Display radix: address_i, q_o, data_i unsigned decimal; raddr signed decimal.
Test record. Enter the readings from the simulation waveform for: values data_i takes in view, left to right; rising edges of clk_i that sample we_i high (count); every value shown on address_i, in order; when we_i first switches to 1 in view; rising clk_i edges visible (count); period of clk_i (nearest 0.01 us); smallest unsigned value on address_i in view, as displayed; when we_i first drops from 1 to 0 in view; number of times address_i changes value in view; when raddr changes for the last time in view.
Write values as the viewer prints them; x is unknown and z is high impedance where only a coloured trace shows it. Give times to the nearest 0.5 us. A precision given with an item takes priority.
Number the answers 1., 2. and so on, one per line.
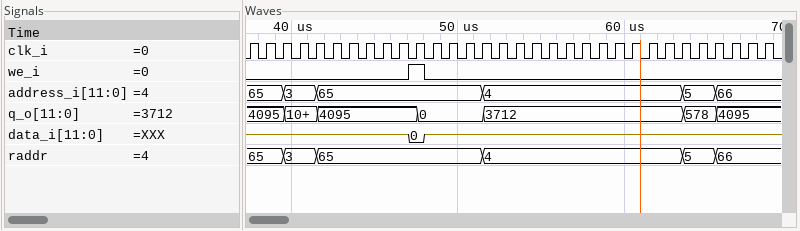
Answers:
1. z, 0, z
2. 1
3. 65, 3, 65, 4, 5, 66
4. 47 us
5. 32
6. 1 us
7. 3
8. 48 us
9. 5
10. 65.5 us
